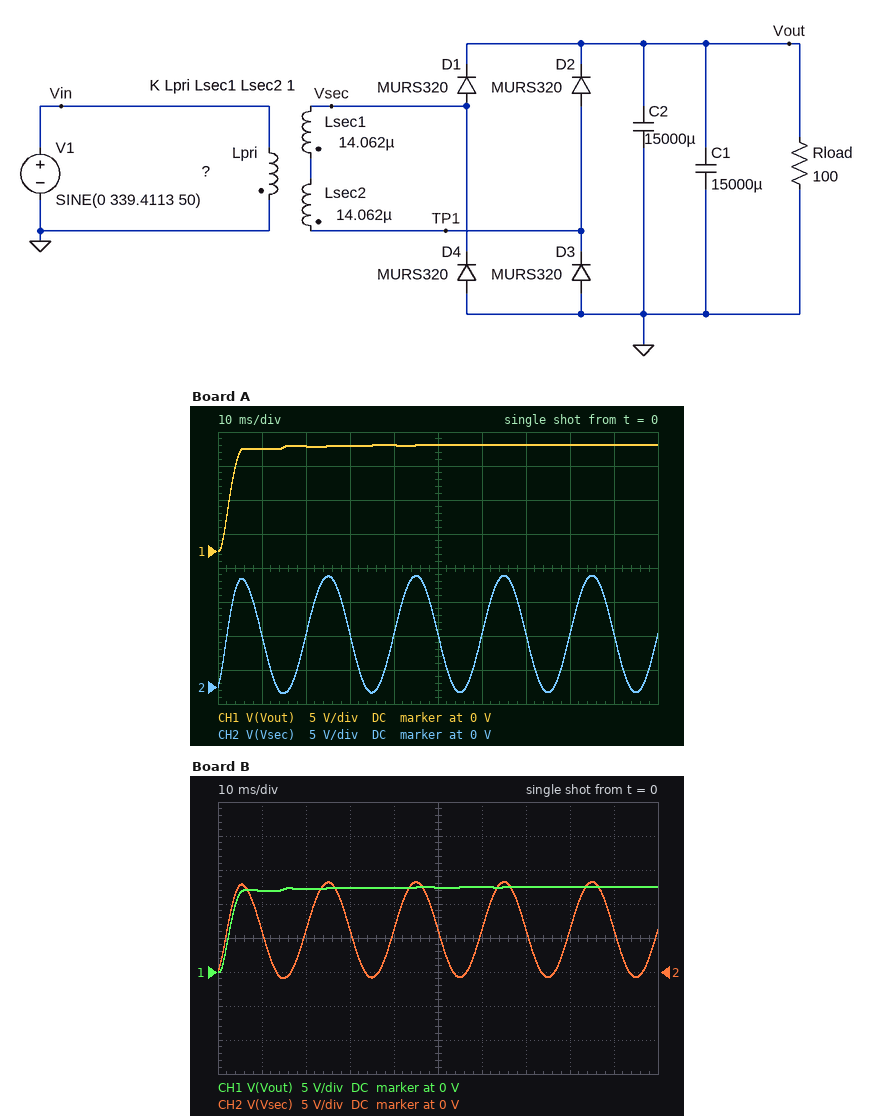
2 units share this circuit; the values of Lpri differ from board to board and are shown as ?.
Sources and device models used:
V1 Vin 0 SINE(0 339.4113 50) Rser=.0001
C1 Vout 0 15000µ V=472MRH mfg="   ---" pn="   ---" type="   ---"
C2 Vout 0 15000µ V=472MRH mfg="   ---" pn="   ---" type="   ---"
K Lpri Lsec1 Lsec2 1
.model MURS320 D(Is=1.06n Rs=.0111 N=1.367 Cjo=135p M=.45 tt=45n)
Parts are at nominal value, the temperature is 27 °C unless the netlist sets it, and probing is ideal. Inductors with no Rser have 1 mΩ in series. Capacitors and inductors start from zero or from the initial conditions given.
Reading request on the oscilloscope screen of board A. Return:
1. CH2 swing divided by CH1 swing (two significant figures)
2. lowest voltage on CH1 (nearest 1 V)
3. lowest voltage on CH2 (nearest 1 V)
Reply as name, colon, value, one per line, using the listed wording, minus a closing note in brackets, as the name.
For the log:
CH2 swing divided by CH1 swing: 1.1
lowest voltage on CH1: 0 V
lowest voltage on CH2: -1 V
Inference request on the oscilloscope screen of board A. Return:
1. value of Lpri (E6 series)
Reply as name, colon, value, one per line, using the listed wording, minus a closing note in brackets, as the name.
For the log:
value of Lpri: 22 mH
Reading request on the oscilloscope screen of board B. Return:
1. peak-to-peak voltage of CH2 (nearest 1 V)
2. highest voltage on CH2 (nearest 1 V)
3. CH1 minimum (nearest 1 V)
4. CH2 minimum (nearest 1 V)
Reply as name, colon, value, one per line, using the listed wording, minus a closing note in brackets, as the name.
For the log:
peak-to-peak voltage of CH2: 14 V
highest voltage on CH2: 13 V
CH1 minimum: 0 V
CH2 minimum: -1 V
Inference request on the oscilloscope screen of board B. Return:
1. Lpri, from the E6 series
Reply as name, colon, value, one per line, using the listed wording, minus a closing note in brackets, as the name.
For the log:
Lpri, from the E6 series: 33 mH
